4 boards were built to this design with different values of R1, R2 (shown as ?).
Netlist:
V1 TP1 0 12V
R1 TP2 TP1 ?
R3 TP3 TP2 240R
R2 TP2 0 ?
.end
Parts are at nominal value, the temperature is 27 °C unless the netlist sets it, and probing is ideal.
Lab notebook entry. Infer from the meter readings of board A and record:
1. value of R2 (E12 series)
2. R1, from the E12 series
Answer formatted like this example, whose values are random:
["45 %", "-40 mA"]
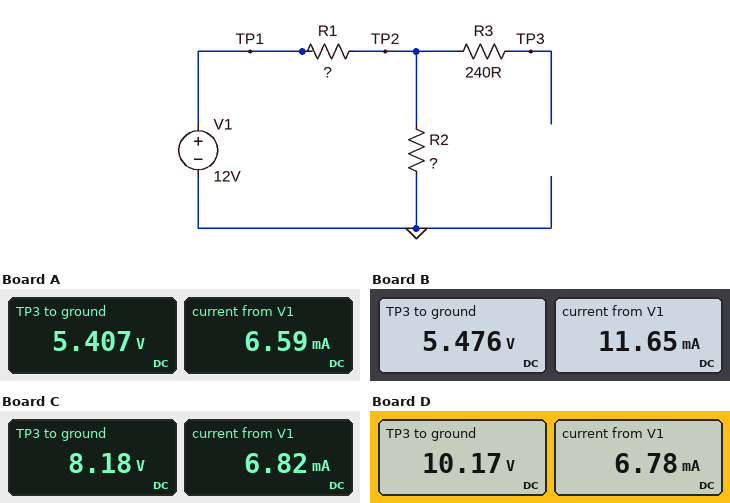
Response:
["820 Ω", "1 kΩ"]
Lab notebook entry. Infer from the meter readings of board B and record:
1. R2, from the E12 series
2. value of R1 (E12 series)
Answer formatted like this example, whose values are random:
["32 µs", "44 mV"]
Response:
["470 Ω", "560 Ω"]
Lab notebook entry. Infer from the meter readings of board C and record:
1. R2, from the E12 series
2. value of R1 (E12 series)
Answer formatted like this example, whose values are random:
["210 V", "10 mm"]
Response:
["1.2 kΩ", "560 Ω"]
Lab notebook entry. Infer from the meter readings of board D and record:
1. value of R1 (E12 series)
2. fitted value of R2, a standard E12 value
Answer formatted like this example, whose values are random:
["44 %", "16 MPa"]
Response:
["270 Ω", "1.5 kΩ"]
